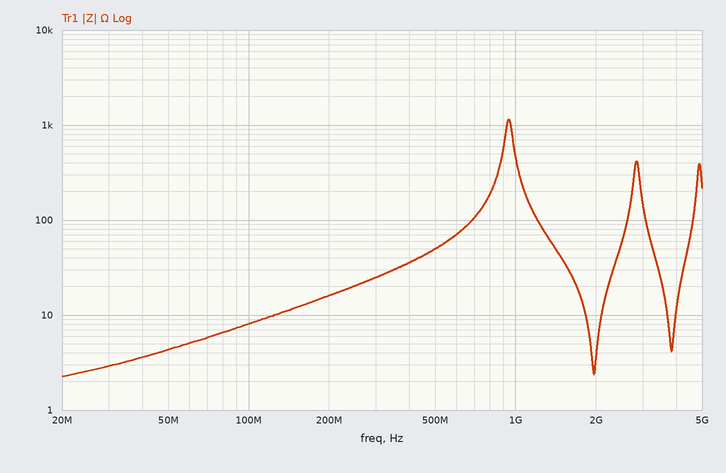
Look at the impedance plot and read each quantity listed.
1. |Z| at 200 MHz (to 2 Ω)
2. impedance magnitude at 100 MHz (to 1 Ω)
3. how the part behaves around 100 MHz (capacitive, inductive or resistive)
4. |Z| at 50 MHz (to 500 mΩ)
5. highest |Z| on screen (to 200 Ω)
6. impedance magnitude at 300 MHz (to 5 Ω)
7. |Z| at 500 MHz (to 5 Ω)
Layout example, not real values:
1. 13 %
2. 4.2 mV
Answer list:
1. 16 Ω
2. 8 Ω
3. inductive
4. 4.5 Ω
5. 1.2 kΩ
6. 25 Ω
7. 50 Ω
